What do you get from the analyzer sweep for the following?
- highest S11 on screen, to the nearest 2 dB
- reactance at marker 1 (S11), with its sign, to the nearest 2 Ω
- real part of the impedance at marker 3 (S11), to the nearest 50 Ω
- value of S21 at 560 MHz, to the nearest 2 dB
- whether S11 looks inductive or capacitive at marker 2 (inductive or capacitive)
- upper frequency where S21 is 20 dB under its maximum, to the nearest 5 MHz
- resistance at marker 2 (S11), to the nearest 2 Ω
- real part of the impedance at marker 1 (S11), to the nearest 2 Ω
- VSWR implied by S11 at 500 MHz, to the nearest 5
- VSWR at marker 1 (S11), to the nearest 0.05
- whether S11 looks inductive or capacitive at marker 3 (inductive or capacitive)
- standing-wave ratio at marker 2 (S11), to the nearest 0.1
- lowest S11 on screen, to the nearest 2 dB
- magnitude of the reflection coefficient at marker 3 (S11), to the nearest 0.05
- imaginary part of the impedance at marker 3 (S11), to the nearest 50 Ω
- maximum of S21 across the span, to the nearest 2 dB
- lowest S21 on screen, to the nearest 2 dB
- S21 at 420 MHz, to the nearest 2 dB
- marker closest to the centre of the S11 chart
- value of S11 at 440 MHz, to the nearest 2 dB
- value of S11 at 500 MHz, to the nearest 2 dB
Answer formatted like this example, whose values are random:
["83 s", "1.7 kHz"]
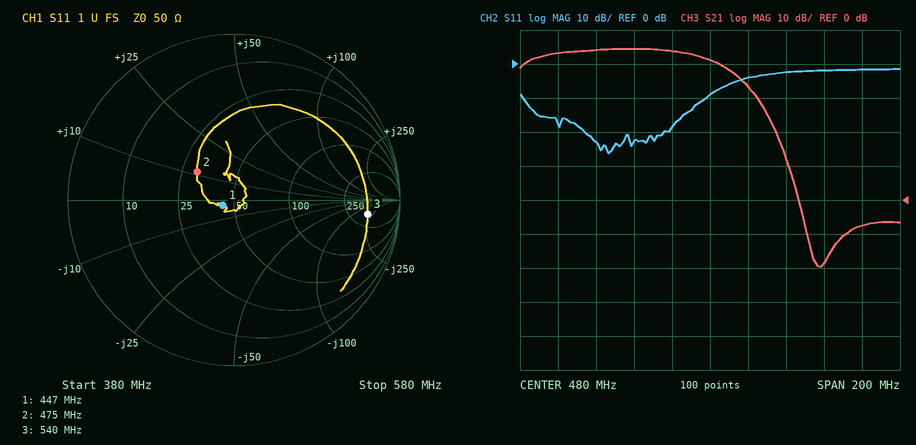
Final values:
["-2 dB", "-2 Ω", "400 Ω", "-8 dB", "inductive", "510 MHz", "30 Ω", "44 Ω", "5", "1.15", "capacitive", "1.8", "-26 dB", "0.80", "-200 Ω", "44 dB", "-20 dB", "44 dB", "marker 1", "-22 dB", "-4 dB"]
